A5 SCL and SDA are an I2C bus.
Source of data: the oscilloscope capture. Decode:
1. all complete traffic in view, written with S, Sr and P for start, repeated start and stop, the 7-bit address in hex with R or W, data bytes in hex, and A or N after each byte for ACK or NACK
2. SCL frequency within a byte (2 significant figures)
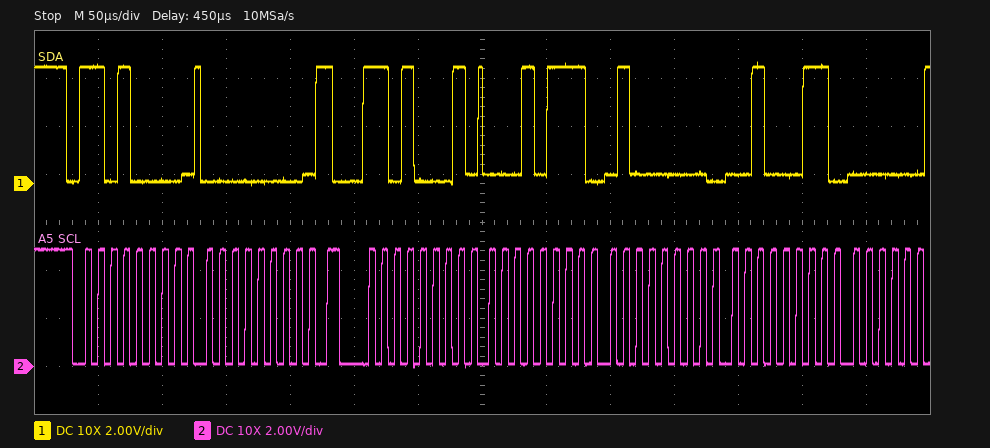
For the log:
S 68W A 00 A Sr 68R A 17 A 40 A 23 A
100 kHz
